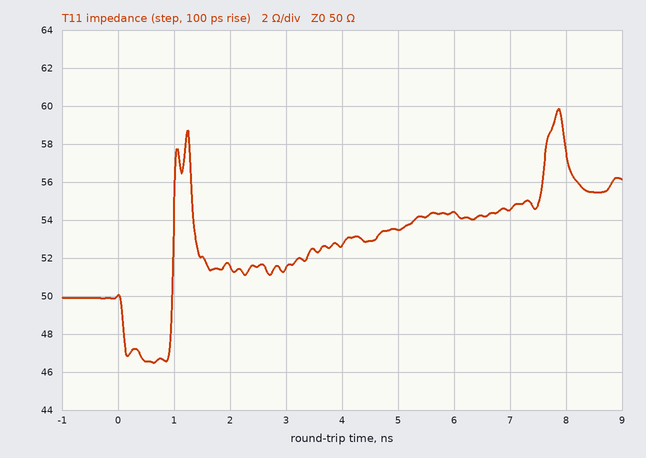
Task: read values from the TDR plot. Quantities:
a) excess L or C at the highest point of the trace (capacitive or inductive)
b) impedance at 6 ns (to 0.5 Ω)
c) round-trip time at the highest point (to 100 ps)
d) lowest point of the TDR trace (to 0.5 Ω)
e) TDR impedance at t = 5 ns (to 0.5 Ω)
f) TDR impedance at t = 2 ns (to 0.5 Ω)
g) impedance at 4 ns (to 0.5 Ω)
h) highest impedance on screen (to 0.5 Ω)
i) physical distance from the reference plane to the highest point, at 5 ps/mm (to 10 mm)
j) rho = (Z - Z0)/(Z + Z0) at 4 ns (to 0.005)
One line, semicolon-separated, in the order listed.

inductive; 54.5 Ω; 7.9 ns; 46.5 Ω; 53.5 Ω; 51.5 Ω; 52.5 Ω; 60.0 Ω; 790 mm; +0.025
